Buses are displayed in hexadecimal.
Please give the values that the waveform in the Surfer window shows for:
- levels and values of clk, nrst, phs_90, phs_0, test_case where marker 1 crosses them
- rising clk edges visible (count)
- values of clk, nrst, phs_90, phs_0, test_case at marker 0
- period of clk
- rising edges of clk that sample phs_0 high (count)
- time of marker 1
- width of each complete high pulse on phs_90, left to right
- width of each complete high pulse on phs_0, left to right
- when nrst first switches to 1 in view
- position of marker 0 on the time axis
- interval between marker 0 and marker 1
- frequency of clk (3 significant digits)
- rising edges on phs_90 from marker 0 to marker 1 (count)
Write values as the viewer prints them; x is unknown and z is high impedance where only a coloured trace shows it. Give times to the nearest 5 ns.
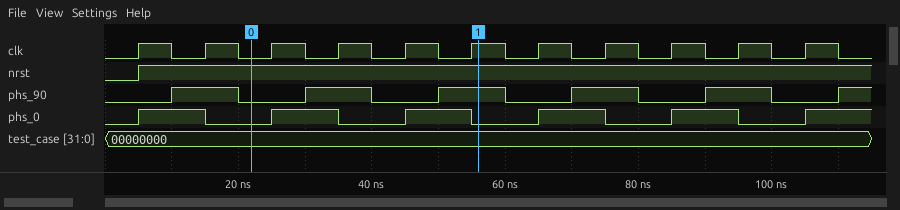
clk=1, nrst=1, phs_90=1, phs_0=0, test_case=00000000
11
clk=0, nrst=1, phs_90=0, phs_0=0, test_case=00000000
10 ns
5
55 ns
10 ns, 10 ns, 10 ns, 10 ns, 10 ns
10 ns, 10 ns, 10 ns, 10 ns, 10 ns
5 ns
20 ns
35 ns
100 MHz
2
